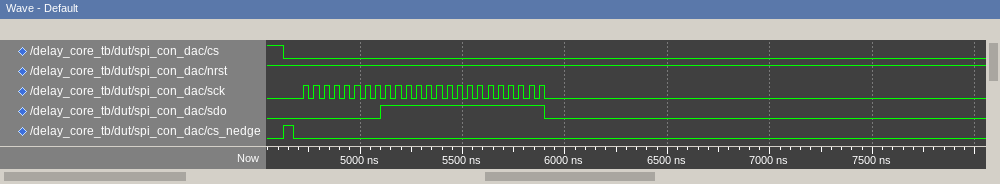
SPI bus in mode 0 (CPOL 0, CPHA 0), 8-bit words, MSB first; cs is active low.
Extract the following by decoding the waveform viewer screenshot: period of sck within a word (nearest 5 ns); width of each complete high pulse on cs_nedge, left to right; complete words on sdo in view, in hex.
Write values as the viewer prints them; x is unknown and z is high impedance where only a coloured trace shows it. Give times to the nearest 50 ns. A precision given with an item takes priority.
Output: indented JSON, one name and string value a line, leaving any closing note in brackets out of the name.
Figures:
{
  "period of sck within a word": "50 ns",
  "width of each complete high pulse on cs_nedge, left to right": "50 ns",
  "complete words on sdo in view, in hex": "00, FF, FF"
}
